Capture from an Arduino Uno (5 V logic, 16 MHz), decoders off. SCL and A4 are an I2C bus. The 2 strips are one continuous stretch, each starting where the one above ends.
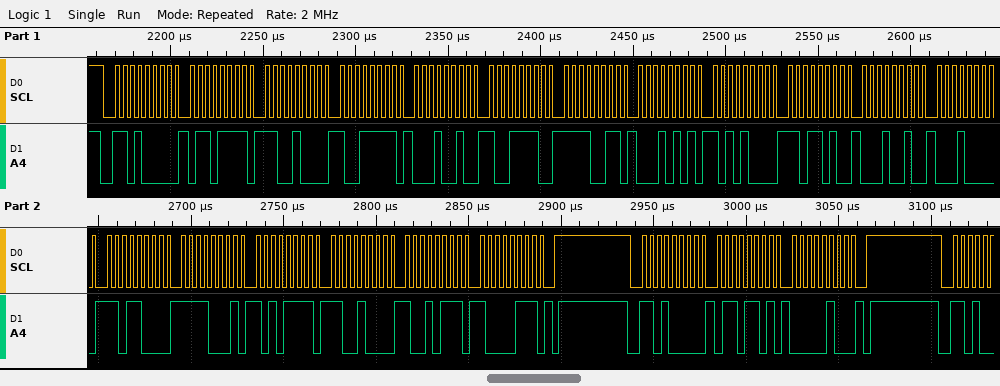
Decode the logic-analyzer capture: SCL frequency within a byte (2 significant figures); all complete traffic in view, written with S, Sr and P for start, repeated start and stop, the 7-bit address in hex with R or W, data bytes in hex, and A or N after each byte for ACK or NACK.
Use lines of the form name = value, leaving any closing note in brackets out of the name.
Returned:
SCL frequency within a byte = 250 kHz
all complete traffic in view, written with S, Sr and P for start, repeated start and stop, the 7-bit address in hex with R or W, data bytes in hex, and A or N after each byte for ACK or NACK = S 68W A 6F A C8 A 9F A 12 A 9E A F3 A 15 A A8 A DA A 12 A 10 A D8 A F1 A AF A C8 A 97 A 87 A P S 68W A 6D A 04 A P
